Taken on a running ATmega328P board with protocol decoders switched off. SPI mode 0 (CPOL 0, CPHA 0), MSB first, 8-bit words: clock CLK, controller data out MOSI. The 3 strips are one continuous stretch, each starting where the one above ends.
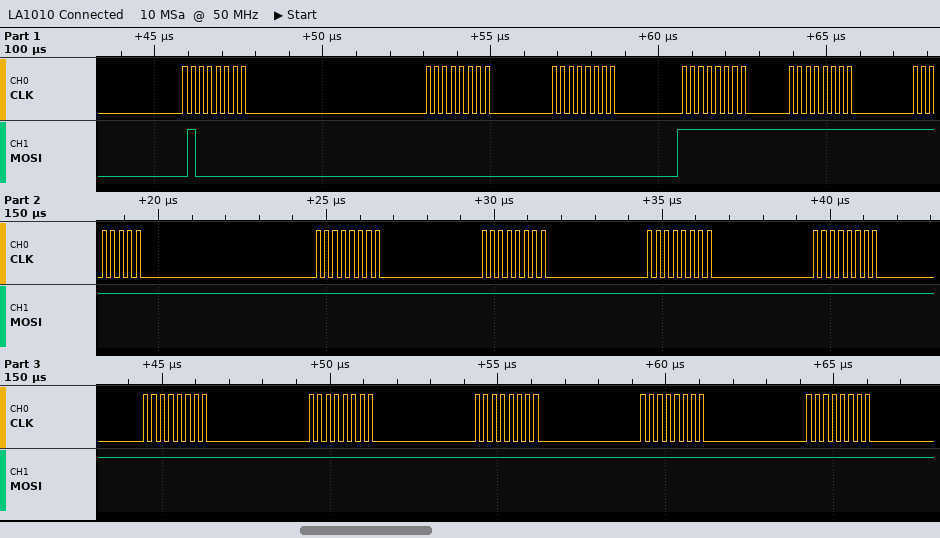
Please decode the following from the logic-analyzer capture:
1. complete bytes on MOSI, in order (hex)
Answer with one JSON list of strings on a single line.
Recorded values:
["40 00 00 FF FF FF FF FF FF FF FF FF FF FF FF"]
